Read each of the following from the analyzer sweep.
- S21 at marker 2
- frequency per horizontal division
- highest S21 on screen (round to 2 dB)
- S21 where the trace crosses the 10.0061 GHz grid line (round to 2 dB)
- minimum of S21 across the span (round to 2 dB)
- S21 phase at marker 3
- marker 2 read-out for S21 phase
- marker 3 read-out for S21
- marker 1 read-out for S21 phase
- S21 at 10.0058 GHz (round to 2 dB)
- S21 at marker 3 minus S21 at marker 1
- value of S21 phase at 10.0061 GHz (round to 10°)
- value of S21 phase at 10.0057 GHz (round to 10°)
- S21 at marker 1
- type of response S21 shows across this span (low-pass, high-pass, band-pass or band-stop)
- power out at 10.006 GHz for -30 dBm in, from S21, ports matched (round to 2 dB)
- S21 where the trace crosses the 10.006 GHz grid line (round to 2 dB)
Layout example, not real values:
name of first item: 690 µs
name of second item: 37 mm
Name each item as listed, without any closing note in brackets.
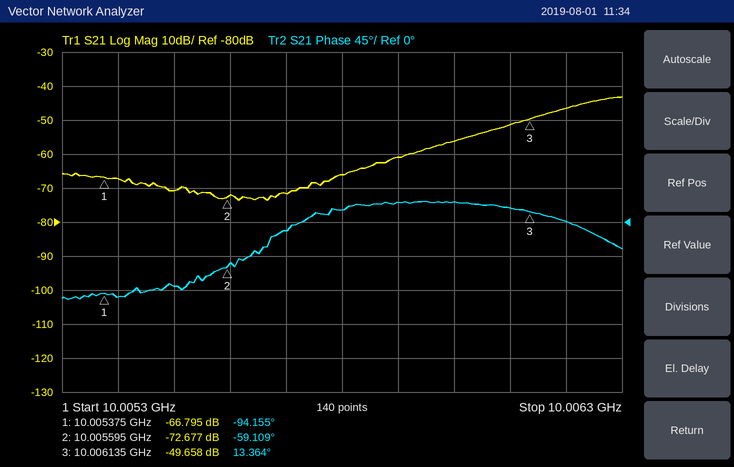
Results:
S21 at marker 2: -72.677 dB
frequency per horizontal division: 100 kHz
highest S21 on screen: -44 dB
S21 where the trace crosses the 10.0061 GHz grid line: -52 dB
minimum of S21 across the span: -74 dB
S21 phase at marker 3: 13.364°
marker 2 read-out for S21 phase: -59.109°
marker 3 read-out for S21: -49.658 dB
marker 1 read-out for S21 phase: -94.155°
S21 at 10.0058 GHz: -66 dB
S21 at marker 3 minus S21 at marker 1: 17.137 dB
value of S21 phase at 10.0061 GHz: 20°
value of S21 phase at 10.0057 GHz: -10°
S21 at marker 1: -66.795 dB
type of response S21 shows across this span: high-pass
power out at 10.006 GHz for -30 dBm in, from S21, ports matched: -86 dBm
S21 where the trace crosses the 10.006 GHz grid line: -56 dB
